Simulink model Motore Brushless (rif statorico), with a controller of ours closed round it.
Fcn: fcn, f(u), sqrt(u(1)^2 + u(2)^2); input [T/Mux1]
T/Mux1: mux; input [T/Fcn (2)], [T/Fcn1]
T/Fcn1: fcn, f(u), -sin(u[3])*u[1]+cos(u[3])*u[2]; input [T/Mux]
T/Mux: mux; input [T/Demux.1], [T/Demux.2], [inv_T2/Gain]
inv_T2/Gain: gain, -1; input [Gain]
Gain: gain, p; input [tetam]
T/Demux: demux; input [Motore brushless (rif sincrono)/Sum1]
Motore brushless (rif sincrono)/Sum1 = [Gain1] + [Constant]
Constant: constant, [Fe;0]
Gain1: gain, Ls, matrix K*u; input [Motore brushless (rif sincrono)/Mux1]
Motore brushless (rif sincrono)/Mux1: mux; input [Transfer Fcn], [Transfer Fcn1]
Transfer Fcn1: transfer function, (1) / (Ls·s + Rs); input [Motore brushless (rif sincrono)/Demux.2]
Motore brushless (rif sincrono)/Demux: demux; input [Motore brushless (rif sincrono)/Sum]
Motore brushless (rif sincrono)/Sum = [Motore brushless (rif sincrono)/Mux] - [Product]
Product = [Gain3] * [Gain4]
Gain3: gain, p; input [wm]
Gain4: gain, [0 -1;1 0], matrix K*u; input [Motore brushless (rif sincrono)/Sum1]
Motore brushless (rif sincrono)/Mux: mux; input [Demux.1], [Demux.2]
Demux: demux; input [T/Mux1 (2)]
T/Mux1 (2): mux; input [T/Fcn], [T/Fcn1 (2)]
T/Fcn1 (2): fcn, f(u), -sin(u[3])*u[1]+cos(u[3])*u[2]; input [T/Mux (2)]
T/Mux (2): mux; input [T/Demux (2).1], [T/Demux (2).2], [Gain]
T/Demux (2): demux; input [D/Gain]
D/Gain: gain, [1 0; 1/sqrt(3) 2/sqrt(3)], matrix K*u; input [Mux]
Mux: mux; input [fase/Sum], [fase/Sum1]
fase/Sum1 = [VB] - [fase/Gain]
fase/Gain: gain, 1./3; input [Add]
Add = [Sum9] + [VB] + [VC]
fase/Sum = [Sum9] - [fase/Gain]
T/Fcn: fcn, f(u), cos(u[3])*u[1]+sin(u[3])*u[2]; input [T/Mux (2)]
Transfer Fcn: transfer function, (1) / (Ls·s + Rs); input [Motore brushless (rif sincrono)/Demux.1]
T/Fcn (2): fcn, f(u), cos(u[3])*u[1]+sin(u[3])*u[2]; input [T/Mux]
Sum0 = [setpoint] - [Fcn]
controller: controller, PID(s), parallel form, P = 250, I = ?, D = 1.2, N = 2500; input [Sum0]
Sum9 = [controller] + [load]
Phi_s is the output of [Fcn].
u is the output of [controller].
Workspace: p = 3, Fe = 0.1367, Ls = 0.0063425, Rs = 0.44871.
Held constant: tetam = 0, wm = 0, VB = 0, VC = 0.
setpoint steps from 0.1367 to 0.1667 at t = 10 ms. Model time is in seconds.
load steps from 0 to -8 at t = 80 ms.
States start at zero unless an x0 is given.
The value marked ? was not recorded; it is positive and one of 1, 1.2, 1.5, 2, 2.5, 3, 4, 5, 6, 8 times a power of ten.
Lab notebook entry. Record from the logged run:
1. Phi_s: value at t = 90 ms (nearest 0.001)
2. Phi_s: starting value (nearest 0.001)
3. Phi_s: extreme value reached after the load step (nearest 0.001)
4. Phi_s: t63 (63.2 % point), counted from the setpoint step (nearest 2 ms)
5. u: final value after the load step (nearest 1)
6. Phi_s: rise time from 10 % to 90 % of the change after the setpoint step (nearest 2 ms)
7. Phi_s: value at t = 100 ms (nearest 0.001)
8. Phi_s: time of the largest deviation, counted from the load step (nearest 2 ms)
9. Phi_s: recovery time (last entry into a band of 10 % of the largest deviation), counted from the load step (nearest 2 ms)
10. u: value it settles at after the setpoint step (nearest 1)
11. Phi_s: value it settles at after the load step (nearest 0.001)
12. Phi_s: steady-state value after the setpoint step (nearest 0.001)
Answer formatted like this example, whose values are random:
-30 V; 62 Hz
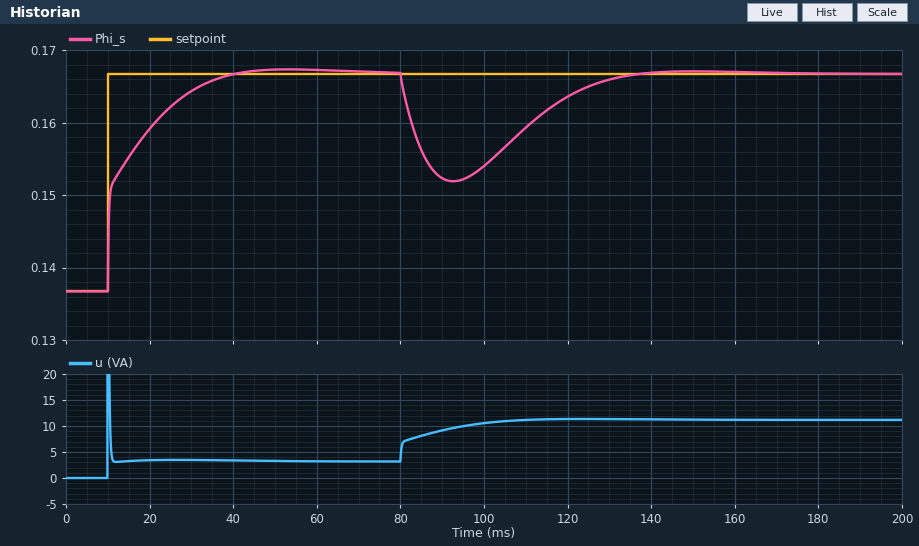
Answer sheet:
0.152; 0.137; 0.152; 6 ms; 11; 18 ms; 0.154; 12 ms; 46 ms; 3; 0.167; 0.167
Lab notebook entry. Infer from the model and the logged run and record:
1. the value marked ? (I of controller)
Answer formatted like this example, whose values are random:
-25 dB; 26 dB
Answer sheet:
20000
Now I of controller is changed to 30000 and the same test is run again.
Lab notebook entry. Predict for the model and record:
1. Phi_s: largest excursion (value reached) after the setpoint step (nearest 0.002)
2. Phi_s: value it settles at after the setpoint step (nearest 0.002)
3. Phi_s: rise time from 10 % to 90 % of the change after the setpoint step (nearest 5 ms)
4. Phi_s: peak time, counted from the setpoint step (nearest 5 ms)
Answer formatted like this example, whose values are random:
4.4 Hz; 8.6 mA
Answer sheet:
0.168; 0.166; 15 ms; 30 ms
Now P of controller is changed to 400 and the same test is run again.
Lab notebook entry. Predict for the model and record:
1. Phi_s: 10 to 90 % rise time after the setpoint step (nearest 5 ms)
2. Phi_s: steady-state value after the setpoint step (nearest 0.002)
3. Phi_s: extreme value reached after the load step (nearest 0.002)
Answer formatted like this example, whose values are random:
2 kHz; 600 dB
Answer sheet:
15 ms; 0.166; 0.154
